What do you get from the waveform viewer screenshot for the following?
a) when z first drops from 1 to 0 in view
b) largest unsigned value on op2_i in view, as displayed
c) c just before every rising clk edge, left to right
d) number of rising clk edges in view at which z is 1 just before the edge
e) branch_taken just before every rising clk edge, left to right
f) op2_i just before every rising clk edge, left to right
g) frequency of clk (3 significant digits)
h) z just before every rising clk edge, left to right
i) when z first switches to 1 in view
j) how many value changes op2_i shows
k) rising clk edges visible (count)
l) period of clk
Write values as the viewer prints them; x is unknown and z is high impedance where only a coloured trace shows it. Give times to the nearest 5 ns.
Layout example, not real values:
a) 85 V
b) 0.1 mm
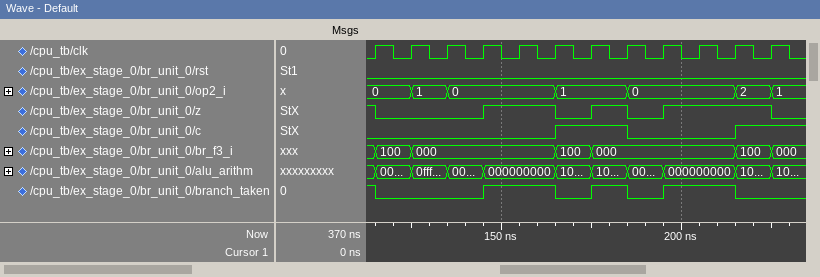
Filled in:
a) 115 ns
b) 2
c) 0 0 0 0 0 0 1 1 0 0 0 1
d) 7
e) 1 0 0 0 1 1 0 1 0 1 1 0
f) 0, 0, 1, 0, 0, 0, 1, 1, 0, 0, 0, 2
g) 100 MHz
h) 1 0 0 0 1 1 0 1 0 1 1 1
i) 145 ns
j) 6
k) 12
l) 10 ns
